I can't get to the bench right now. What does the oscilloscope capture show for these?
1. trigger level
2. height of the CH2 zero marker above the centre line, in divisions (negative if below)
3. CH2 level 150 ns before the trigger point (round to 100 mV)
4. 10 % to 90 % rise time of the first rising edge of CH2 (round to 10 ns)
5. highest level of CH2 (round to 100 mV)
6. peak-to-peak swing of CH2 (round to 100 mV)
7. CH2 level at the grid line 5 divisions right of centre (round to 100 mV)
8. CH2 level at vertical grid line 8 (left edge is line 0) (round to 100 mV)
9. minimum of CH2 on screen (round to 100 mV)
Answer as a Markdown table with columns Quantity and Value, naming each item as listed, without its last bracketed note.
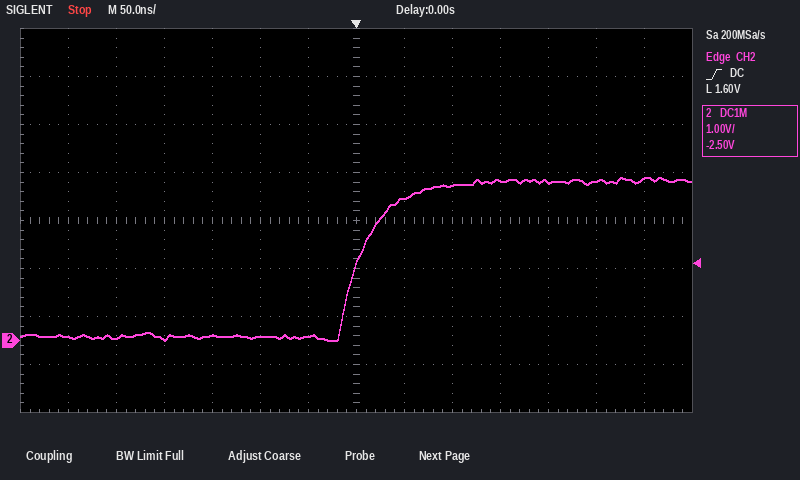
| Quantity | Value |
|---|---|
| trigger level | 1.60 V |
| height of the CH2 zero marker above the centre line, in divisions | -2.5 div |
| CH2 level 150 ns before the trigger point | 100 mV |
| 10 % to 90 % rise time of the first rising edge of CH2 | 70 ns |
| highest level of CH2 | 3.4 V |
| peak-to-peak swing of CH2 | 3.4 V |
| CH2 level at the grid line 5 divisions right of centre | 3.3 V |
| CH2 level at vertical grid line 8 (left edge is line 0) | 3.0 V |
| minimum of CH2 on screen | 0.0 V |
